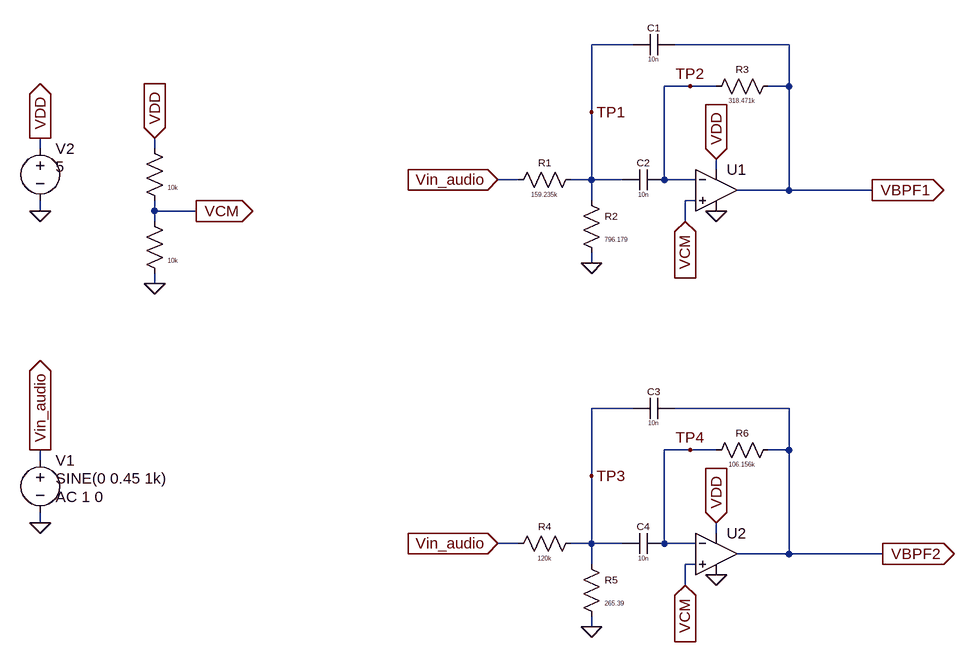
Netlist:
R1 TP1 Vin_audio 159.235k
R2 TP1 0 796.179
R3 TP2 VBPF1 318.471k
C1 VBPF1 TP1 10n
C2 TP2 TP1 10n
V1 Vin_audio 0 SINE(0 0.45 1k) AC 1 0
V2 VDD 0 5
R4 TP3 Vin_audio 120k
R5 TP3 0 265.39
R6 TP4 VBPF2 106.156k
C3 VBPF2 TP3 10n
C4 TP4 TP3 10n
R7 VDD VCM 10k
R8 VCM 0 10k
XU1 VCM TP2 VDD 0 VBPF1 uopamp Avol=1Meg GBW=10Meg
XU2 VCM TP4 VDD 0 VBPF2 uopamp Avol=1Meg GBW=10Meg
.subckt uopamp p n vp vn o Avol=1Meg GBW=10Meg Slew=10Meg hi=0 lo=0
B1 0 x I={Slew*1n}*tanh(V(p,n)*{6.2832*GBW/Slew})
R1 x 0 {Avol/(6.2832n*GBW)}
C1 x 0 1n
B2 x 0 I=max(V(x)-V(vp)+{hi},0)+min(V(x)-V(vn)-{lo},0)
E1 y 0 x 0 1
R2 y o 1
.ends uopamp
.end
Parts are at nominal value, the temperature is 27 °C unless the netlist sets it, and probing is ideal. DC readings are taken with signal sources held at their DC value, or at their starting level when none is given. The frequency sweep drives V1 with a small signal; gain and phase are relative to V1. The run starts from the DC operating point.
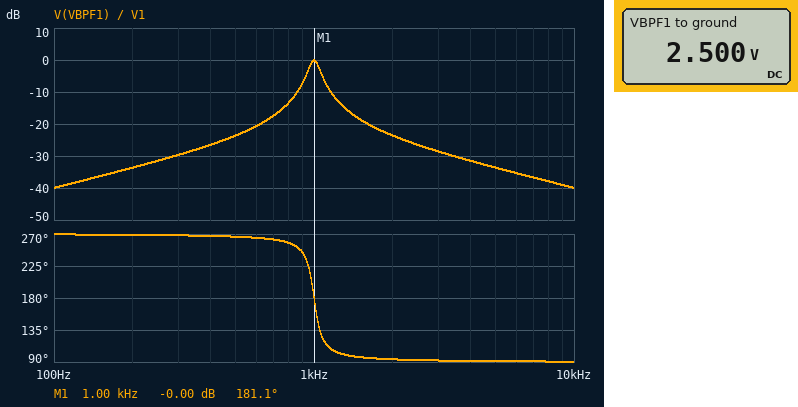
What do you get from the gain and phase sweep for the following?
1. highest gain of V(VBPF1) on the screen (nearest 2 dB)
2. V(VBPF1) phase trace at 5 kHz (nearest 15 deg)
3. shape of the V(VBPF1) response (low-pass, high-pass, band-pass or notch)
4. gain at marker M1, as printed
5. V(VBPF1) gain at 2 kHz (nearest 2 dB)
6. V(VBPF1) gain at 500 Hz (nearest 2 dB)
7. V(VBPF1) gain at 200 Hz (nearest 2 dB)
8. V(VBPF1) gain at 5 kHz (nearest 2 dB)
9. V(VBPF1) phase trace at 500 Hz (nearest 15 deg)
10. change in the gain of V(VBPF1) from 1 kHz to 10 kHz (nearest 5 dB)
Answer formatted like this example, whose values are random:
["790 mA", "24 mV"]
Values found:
["0 dB", "90 deg", "band-pass", "-0.00 dB", "-24 dB", "-24 dB", "-34 dB", "-34 dB", "270 deg", "-40 dB"]
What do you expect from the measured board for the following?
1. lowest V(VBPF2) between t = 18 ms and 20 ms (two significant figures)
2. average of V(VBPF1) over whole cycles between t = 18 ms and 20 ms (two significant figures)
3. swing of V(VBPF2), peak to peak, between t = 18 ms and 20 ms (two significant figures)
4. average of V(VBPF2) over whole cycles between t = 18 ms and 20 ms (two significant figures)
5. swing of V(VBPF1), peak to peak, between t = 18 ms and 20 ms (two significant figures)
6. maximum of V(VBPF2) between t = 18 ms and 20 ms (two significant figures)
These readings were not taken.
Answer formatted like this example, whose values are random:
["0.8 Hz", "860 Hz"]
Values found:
["2.5 V", "2.5 V", "15 mV", "2.5 V", "900 mV", "2.5 V"]
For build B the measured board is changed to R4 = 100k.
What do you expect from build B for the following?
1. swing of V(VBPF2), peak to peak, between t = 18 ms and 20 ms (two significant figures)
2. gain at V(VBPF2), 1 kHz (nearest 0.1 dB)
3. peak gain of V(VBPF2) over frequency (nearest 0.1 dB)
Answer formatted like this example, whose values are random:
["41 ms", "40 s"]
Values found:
["18 mV", "-34.0 dB", "-5.5 dB"]
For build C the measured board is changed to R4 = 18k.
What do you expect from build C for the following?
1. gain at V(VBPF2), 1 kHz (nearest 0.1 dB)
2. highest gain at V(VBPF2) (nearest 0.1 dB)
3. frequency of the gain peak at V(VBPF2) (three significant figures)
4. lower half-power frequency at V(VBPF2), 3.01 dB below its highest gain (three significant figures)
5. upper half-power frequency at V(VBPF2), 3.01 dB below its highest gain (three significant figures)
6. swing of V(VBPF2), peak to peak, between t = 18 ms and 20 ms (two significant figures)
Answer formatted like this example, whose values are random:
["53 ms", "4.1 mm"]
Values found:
["-19.3 dB", "9.4 dB", "3.01 kHz", "2.87 kHz", "3.16 kHz", "98 mV"]
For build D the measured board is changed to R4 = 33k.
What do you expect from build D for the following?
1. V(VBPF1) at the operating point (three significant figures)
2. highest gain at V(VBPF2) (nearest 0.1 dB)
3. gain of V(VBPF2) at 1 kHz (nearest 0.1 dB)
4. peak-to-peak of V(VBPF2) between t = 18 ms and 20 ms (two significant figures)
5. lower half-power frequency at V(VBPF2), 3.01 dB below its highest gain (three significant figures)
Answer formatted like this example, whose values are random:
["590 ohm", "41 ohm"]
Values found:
["2.50 V", "4.1 dB", "-24.5 dB", "54 mV", "2.86 kHz"]
